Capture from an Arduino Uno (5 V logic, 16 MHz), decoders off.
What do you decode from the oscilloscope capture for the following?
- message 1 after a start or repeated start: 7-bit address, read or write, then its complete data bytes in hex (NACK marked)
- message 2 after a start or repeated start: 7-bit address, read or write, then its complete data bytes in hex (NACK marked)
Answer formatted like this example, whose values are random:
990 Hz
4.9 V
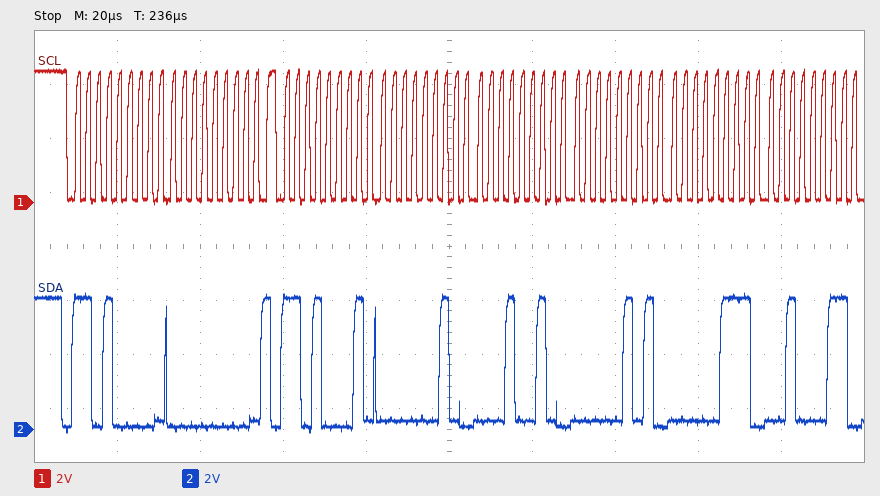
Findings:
0x68 write: 00
0x68 read: 02 12 05 07 23
